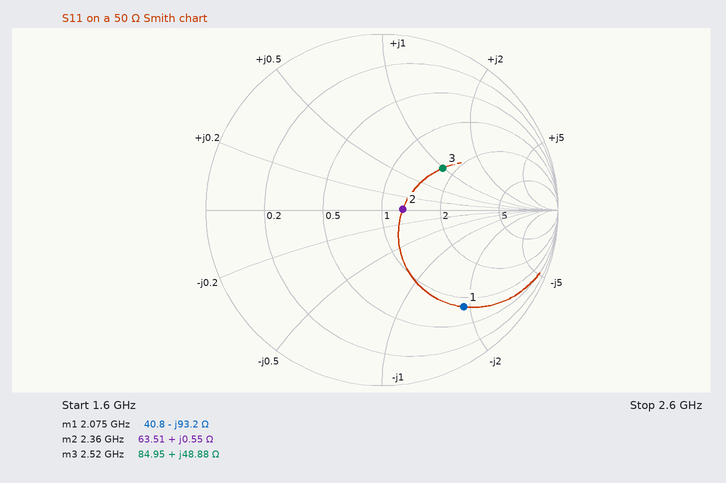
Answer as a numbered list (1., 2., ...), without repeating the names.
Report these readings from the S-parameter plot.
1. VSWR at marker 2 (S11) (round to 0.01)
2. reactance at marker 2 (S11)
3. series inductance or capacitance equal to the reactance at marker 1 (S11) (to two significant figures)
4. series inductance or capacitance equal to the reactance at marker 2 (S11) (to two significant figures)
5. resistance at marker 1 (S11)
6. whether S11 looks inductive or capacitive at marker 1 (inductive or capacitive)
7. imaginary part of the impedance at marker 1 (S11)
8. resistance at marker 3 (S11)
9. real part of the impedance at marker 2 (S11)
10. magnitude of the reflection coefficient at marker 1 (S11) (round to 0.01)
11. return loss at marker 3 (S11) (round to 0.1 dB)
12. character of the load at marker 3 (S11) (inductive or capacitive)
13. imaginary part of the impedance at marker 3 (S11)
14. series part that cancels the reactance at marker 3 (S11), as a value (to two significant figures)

1. 1.27
2. +0.55 Ω
3. 820 fF
4. 37 pH
5. 40.8 Ω
6. capacitive
7. -93.2 Ω
8. 84.95 Ω
9. 63.51 Ω
10. 0.72
11. 7.6 dB
12. inductive
13. +48.88 Ω
14. 1.3 pF
